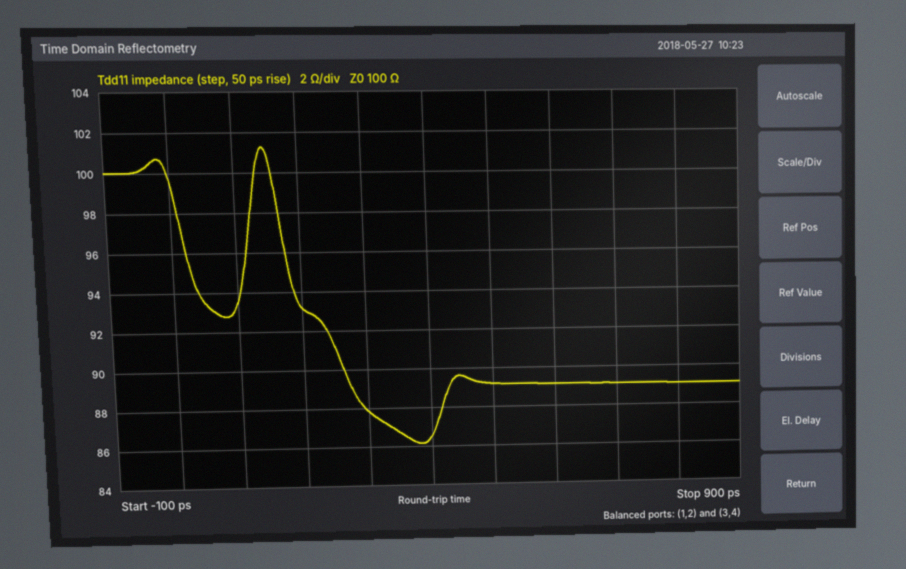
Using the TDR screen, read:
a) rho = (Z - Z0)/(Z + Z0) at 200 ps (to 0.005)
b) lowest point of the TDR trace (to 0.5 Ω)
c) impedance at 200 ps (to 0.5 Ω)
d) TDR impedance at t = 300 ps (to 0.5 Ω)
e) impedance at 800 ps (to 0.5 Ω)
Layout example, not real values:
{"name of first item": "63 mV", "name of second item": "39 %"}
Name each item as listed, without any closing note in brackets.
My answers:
{"rho = (Z - Z0)/(Z + Z0) at 200 ps": "-0.035", "lowest point of the TDR trace": "86.0 Ω", "impedance at 200 ps": "93.0 Ω", "TDR impedance at t = 300 ps": "88.0 Ω", "impedance at 800 ps": "89.0 Ω"}
